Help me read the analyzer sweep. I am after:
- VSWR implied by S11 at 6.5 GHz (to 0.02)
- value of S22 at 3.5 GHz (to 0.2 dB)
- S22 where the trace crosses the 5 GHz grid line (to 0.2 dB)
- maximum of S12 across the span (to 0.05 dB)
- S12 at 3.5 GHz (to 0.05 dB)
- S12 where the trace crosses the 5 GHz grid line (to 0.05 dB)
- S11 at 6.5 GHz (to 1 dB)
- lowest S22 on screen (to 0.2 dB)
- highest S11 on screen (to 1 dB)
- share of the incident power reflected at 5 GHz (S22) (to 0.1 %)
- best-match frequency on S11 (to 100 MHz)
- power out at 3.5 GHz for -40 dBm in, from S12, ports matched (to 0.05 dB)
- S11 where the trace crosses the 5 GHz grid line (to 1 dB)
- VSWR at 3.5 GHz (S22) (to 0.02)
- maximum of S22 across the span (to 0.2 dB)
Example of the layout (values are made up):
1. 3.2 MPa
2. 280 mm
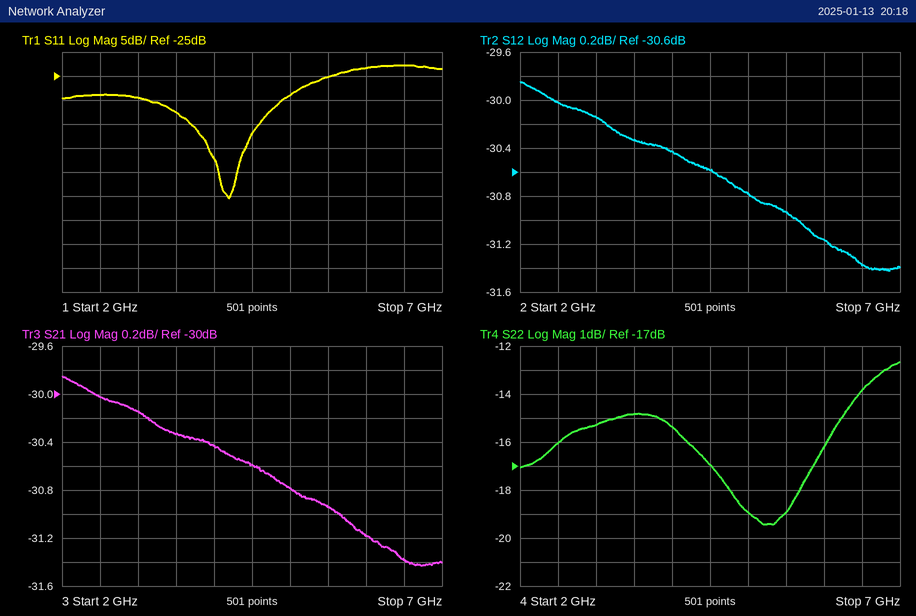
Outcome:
1. 1.16
2. -14.8 dB
3. -19.0 dB
4. -29.85 dB
5. -30.35 dB
6. -30.80 dB
7. -23 dB
8. -19.4 dB
9. -23 dB
10. 1.3 %
11. 4.2 GHz
12. -70.35 dBm
13. -29 dB
14. 1.44
15. -12.6 dB
